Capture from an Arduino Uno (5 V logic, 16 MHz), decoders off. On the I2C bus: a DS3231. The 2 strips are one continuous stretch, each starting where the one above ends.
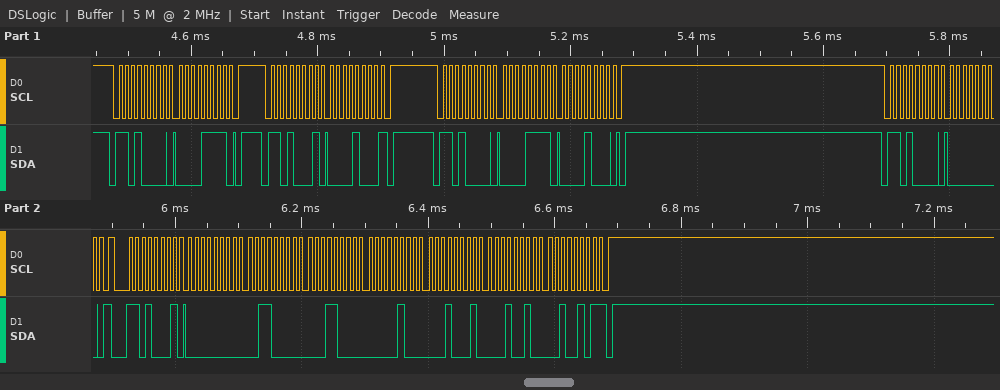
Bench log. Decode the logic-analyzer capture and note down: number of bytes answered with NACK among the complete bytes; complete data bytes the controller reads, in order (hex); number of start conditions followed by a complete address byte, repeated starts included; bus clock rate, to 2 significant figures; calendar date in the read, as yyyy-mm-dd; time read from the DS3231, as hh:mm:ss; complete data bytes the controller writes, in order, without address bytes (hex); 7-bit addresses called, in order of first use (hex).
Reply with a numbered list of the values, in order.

1. 2
2. 08 00 30 18 04 11 12 25
3. 5
4. 100 kHz
5. 2025-12-11
6. 18:30:00
7. 0F 0F 08 00
8. 0x68
